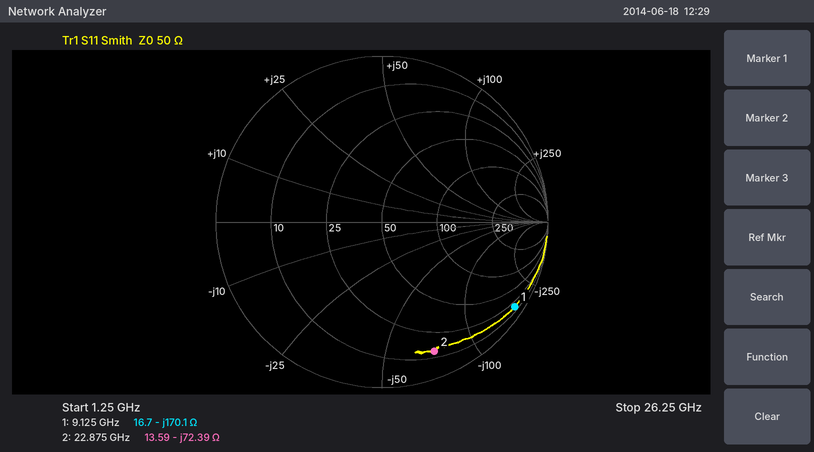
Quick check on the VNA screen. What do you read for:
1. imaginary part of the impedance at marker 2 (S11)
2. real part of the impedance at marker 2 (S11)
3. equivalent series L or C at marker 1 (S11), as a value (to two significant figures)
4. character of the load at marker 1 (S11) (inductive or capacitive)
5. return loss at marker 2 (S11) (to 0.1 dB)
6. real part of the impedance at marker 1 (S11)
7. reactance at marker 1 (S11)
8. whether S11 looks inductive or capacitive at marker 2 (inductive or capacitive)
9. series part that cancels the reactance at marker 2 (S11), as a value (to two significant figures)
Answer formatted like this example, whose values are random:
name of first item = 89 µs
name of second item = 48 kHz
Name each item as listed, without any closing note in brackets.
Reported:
imaginary part of the impedance at marker 2 = -72.39 Ω
real part of the impedance at marker 2 = 13.59 Ω
equivalent series L or C at marker 1 (S11), as a value = 100 fF
character of the load at marker 1 (S11) = capacitive
return loss at marker 2 (S11) = 1.5 dB
real part of the impedance at marker 1 = 16.7 Ω
reactance at marker 1 = -170.1 Ω
whether S11 looks inductive or capacitive at marker 2 = capacitive
series part that cancels the reactance at marker 2 (S11), as a value = 500 pH
